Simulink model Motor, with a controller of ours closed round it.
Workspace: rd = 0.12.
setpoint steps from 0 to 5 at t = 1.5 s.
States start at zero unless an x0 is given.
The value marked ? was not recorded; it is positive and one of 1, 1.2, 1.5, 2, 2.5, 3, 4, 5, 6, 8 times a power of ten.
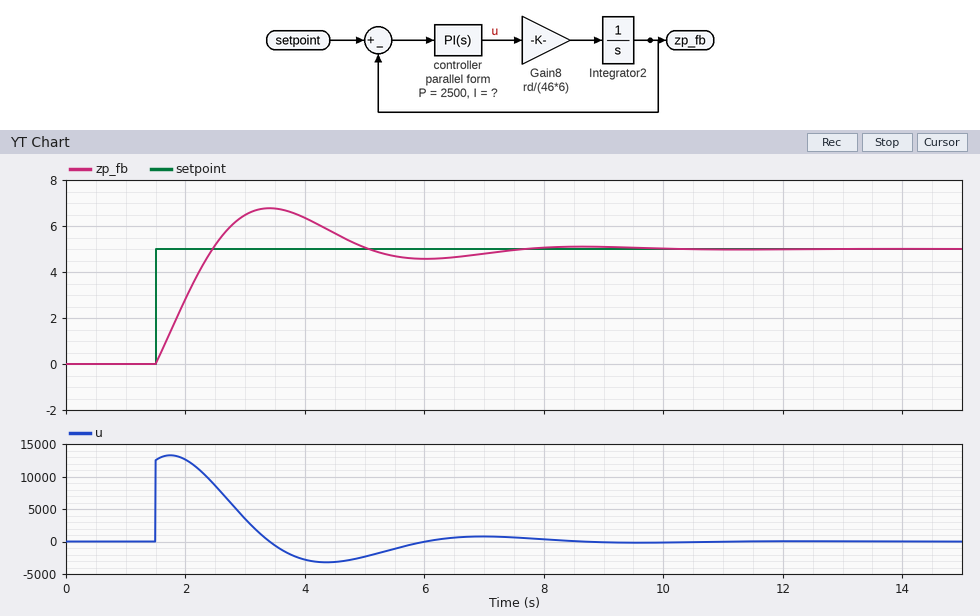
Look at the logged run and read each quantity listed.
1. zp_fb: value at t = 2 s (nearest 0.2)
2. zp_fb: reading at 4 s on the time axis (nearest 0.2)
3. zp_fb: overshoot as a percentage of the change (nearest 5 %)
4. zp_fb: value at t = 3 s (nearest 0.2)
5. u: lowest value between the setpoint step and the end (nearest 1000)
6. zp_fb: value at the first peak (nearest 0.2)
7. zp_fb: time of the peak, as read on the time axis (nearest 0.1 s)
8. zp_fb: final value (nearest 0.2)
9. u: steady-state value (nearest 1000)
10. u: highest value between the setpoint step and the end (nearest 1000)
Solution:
2.8
6.4
35 %
6.4
-3000
6.8
3.4 s
5.0
0
13000
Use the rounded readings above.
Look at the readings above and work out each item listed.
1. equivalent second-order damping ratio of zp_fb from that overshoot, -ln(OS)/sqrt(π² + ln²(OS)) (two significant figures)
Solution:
0.32
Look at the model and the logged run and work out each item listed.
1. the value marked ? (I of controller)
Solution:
4000
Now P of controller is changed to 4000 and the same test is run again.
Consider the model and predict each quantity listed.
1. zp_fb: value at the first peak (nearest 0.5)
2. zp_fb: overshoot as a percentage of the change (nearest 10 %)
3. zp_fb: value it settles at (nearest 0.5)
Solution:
6.0
20 %
5.0
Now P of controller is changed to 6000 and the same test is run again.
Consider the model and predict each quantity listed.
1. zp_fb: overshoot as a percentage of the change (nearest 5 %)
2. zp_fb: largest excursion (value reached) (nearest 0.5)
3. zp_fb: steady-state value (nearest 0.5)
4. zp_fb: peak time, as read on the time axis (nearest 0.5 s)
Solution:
15 %
5.5
5.0
3.0 s
